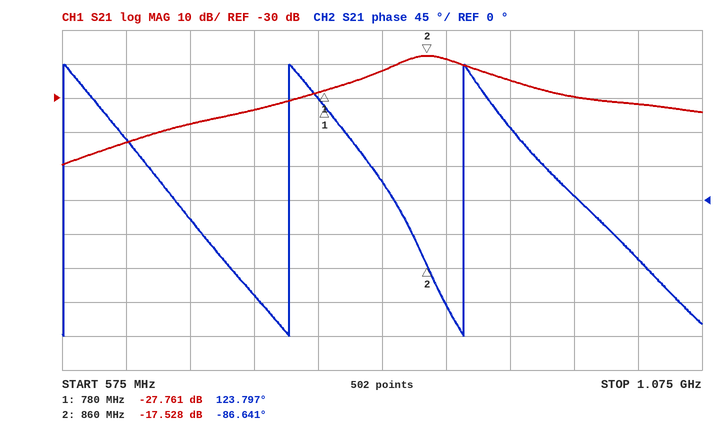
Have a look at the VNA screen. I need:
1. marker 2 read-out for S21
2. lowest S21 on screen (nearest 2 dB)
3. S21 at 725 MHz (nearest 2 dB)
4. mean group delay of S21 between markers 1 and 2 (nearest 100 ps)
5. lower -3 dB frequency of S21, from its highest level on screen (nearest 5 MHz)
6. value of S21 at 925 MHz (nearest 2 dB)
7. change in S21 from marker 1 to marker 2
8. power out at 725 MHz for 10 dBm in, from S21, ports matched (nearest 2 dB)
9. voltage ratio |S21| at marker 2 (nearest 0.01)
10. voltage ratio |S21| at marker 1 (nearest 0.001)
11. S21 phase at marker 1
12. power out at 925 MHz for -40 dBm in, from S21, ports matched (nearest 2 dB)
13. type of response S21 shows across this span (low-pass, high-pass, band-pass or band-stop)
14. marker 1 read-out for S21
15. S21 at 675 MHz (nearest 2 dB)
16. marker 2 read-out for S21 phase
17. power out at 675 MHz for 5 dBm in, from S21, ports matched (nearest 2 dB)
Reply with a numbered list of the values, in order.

1. -17.528 dB
2. -50 dB
3. -34 dB
4. 7.3 ns
5. 835 MHz
6. -24 dB
7. 10.233 dB
8. -24 dBm
9. 0.13
10. 0.041
11. 123.797°
12. -64 dBm
13. band-pass
14. -27.761 dB
15. -38 dB
16. -86.641°
17. -32 dBm
